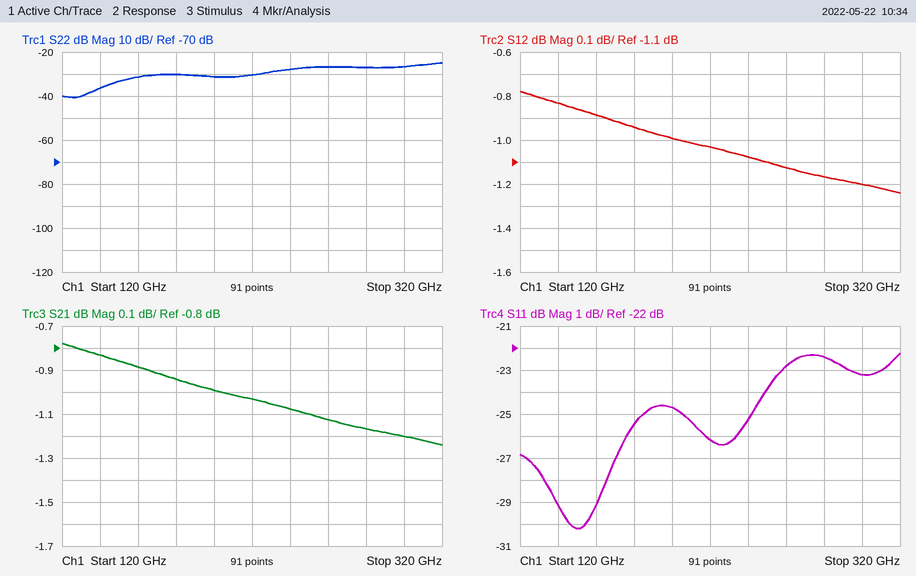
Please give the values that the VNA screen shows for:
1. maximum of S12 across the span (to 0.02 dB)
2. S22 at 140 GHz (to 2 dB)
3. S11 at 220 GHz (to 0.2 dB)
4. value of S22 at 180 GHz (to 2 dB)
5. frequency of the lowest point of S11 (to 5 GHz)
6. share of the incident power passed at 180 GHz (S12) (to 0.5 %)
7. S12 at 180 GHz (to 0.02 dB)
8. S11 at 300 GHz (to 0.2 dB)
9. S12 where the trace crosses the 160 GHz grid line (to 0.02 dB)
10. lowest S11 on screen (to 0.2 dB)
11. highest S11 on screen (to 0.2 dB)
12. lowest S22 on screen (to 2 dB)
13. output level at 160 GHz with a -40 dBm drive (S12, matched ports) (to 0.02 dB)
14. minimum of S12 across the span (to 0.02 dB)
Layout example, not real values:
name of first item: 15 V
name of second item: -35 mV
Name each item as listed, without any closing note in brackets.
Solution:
maximum of S12 across the span: -0.78 dB
S22 at 140 GHz: -36 dB
S11 at 220 GHz: -26.2 dB
value of S22 at 180 GHz: -30 dB
frequency of the lowest point of S11: 150 GHz
share of the incident power passed at 180 GHz (S12): 80.5 %
S12 at 180 GHz: -0.94 dB
S11 at 300 GHz: -23.2 dB
S12 where the trace crosses the 160 GHz grid line: -0.88 dB
lowest S11 on screen: -30.2 dB
highest S11 on screen: -22.2 dB
lowest S22 on screen: -40 dB
output level at 160 GHz with a -40 dBm drive (S12, matched ports): -40.88 dBm
minimum of S12 across the span: -1.24 dB
